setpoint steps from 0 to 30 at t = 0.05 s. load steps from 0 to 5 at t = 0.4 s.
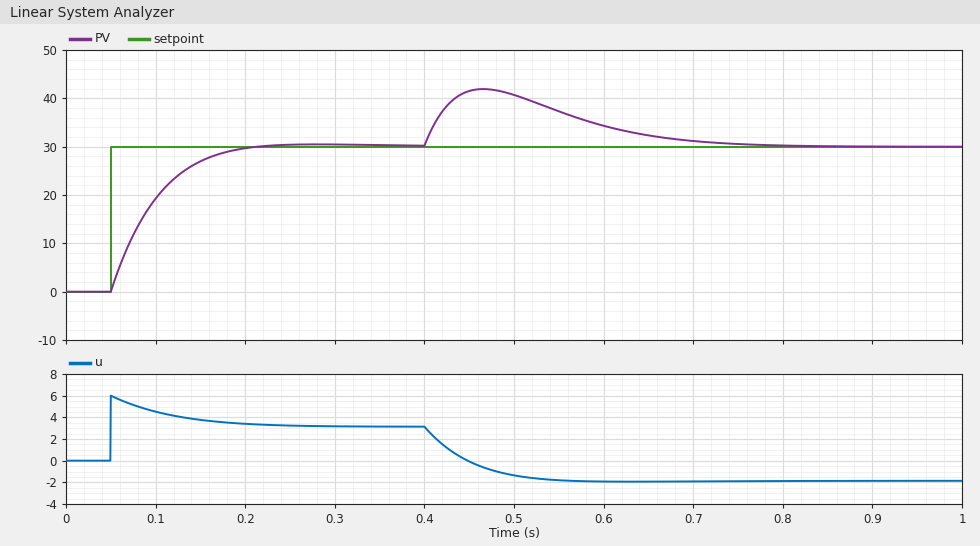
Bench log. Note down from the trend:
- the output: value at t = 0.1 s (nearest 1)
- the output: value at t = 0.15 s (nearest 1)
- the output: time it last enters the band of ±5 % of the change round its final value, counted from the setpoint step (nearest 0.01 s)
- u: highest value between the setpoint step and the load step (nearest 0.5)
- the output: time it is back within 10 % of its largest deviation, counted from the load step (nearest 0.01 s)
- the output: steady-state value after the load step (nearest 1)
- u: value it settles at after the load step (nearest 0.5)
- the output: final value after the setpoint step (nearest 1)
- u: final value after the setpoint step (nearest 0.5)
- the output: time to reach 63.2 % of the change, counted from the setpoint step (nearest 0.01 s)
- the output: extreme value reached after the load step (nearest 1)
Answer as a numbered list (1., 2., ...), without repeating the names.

1. 19
2. 27
3. 0.12 s
4. 6.0
5. 0.30 s
6. 30
7. -2.0
8. 30
9. 3.0
10. 0.05 s
11. 42
